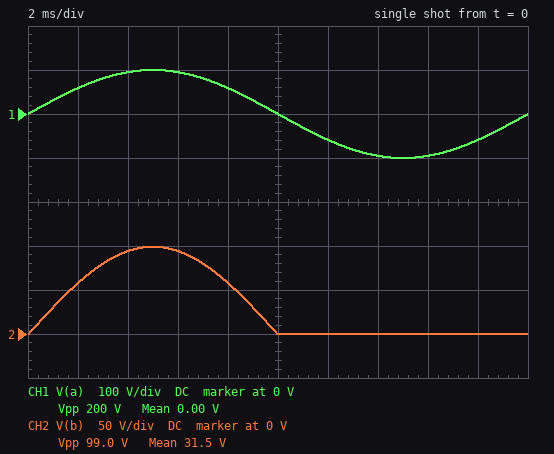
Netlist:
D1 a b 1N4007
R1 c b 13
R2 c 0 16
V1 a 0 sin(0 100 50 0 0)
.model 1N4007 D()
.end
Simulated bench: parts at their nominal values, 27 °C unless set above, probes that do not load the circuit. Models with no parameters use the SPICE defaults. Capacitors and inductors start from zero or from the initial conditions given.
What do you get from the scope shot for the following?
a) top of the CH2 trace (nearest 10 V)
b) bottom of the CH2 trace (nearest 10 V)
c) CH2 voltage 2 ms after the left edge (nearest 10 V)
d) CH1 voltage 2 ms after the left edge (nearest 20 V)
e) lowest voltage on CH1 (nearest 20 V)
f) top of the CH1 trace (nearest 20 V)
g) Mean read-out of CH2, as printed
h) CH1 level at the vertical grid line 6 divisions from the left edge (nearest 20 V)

100 V
0 V
60 V
60 V
-100 V
100 V
31.5 V
-60 V
